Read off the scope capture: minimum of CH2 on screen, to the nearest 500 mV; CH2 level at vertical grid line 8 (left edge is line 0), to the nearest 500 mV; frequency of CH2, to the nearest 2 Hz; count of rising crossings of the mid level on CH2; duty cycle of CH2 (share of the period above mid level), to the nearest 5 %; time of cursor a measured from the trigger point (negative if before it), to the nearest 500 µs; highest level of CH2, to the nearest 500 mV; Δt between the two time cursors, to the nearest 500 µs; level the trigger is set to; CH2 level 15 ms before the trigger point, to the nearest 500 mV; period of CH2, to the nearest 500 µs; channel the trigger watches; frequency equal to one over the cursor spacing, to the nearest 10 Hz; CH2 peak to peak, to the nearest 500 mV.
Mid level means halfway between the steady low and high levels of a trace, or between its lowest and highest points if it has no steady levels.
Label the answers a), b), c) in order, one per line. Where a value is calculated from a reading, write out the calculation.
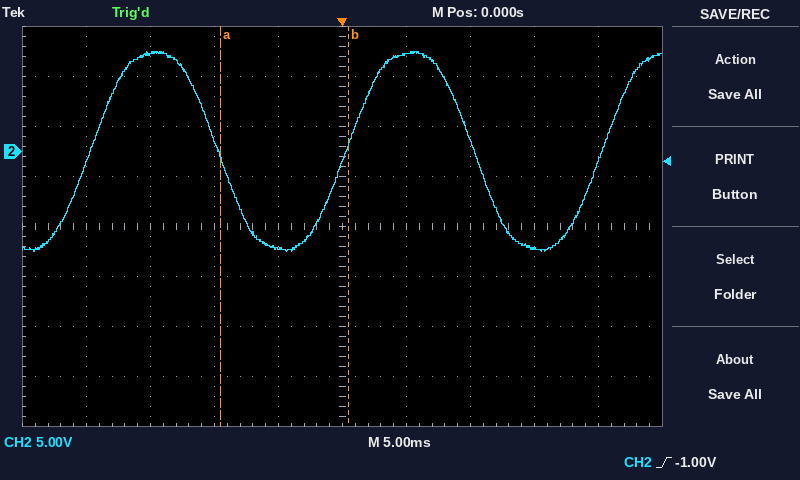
a) -10.0 V
b) -9.5 V
c) 1 / 20.0 ms ≈ 50 Hz
d) 3
e) 50 %
f) -9.5 ms
g) 10.0 V
h) 10.0 ms
i) -1.00 V
j) 10.0 V
k) 20.0 ms
l) CH2
m) 1 / 10.0 ms ≈ 100 Hz
n) 10.0 V − (-10.0 V) = 20.0 V
